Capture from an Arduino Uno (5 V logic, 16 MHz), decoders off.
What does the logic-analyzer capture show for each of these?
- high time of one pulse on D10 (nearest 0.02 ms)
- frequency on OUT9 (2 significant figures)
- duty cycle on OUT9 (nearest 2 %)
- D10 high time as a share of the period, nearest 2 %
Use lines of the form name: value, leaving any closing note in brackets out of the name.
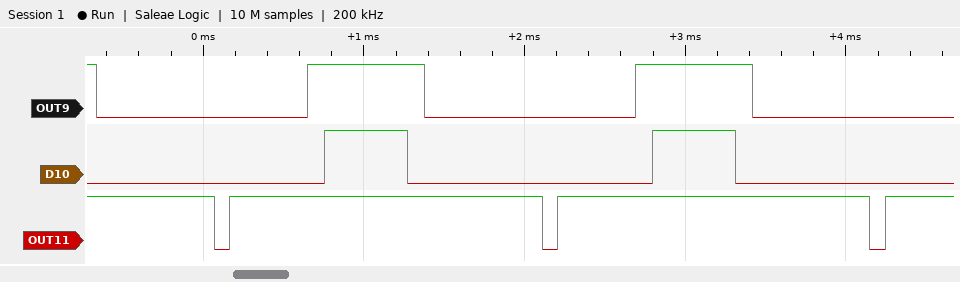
high time of one pulse on D10: 0.52 ms
frequency on OUT9: 490 Hz
duty cycle on OUT9: 36 %
D10 high time as a share of the period, nearest 2 %: 26 %
